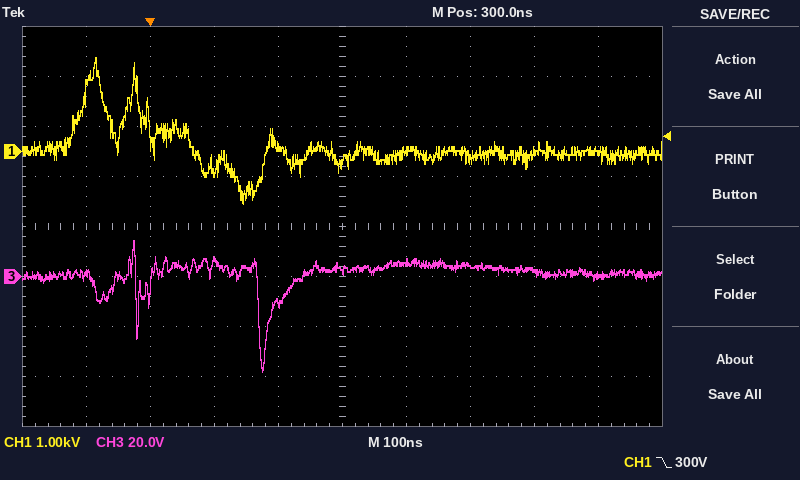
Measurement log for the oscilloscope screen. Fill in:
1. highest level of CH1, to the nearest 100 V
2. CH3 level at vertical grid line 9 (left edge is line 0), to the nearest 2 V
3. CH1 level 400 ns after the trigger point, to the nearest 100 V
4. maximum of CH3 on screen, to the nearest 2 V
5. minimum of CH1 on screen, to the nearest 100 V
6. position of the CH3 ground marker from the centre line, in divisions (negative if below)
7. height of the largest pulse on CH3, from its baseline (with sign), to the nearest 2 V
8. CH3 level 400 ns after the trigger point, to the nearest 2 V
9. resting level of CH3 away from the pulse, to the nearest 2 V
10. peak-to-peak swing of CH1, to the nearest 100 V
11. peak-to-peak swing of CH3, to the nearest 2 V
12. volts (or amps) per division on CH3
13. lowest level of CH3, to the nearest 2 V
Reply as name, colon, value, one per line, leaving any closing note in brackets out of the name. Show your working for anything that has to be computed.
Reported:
highest level of CH1, to the nearest 100 V: 1.9 kV
CH3 level at vertical grid line 9 (left edge is line 0), to the nearest 2 V: 0 V
CH1 level 400 ns after the trigger point, to the nearest 100 V: 0.0 kV
maximum of CH3 on screen, to the nearest 2 V: 14 V
minimum of CH1 on screen, to the nearest 100 V: -1.0 kV
position of the CH3 ground marker from the centre line, in divisions: -1.0 div
height of the largest pulse on CH3, from its baseline (with sign), to the nearest 2 V: -38 V − (2 V) = -40 V
CH3 level 400 ns after the trigger point, to the nearest 2 V: 6 V
resting level of CH3 away from the pulse, to the nearest 2 V: 2 V
peak-to-peak swing of CH1, to the nearest 100 V: 1.9 kV − (-1.0 kV) = 2.9 kV
peak-to-peak swing of CH3, to the nearest 2 V: 14 V − (-38 V) = 52 V
volts (or amps) per division on CH3: 20 V
lowest level of CH3, to the nearest 2 V: -38 V
